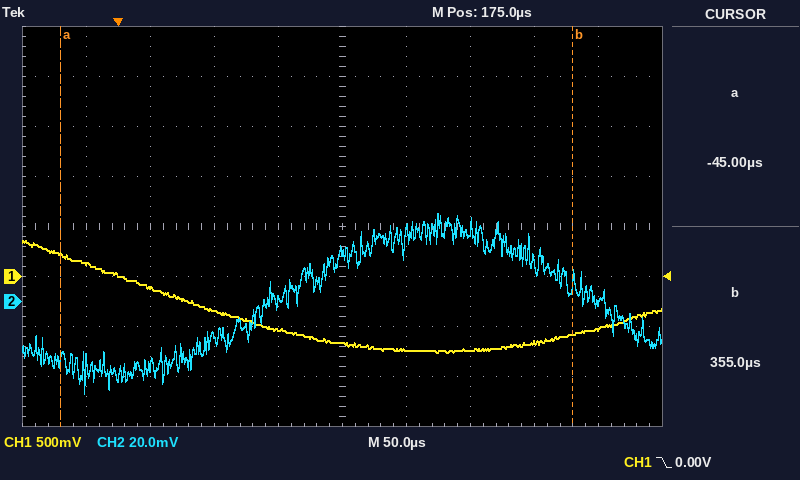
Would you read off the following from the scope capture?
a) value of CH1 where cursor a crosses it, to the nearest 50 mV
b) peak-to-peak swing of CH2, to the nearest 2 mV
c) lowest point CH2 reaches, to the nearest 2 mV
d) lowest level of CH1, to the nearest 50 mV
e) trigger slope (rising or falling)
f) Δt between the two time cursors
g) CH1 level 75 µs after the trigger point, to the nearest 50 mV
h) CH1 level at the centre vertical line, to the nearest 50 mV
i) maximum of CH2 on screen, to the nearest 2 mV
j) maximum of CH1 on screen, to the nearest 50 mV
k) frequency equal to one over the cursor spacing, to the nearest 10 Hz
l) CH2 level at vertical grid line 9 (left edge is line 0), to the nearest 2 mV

200 mV
72 mV
-36 mV
-750 mV
falling
400 µs
-350 mV
-650 mV
36 mV
350 mV
2.50 kHz
0 mV
